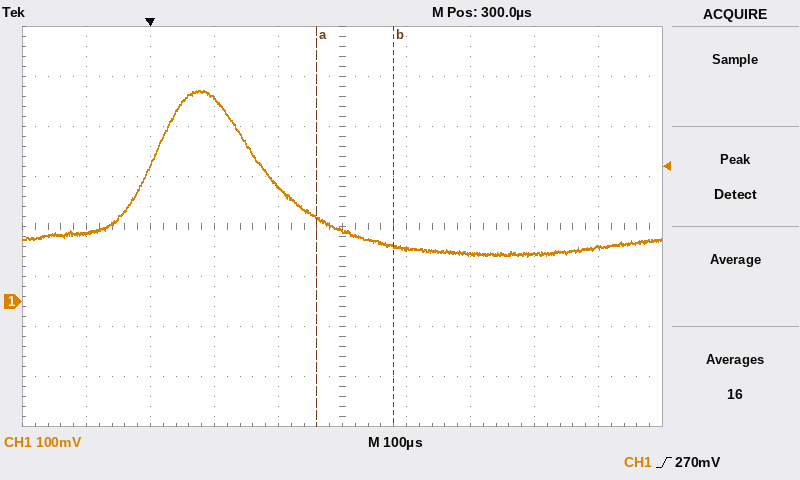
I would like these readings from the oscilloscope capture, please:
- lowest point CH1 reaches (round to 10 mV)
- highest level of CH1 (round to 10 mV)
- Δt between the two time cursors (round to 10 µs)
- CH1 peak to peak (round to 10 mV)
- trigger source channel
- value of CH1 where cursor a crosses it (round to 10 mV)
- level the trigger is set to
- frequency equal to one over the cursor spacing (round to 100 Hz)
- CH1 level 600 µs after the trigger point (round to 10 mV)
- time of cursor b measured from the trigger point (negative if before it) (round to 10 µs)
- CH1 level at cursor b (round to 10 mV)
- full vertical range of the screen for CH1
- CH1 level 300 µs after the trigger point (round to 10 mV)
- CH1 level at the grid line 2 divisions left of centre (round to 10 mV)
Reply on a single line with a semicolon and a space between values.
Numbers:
90 mV; 420 mV; 120 µs; 330 mV; CH1; 170 mV; 270 mV; 8.3 kHz; 100 mV; +380 µs; 110 mV; 800 mV; 140 mV; 410 mV
